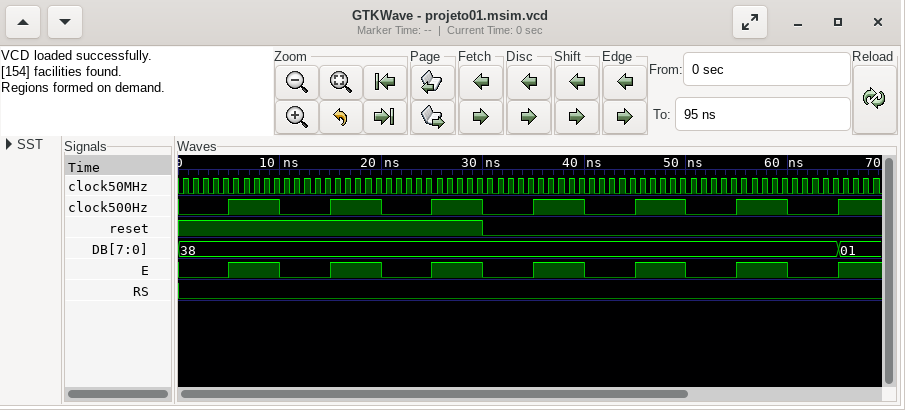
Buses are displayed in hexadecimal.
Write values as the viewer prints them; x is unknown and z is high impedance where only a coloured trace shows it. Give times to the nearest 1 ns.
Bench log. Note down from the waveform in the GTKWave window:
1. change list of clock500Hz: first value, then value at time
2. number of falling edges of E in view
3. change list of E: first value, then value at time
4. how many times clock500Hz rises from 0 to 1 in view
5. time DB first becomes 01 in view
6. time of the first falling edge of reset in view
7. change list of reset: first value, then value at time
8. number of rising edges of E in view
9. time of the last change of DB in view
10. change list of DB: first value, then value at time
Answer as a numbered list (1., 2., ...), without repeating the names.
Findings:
1. 0, 1 at 5 ns, 0 at 10 ns, 1 at 15 ns, 0 at 20 ns, 1 at 25 ns, 0 at 30 ns, 1 at 35 ns, 0 at 40 ns, 1 at 45 ns, 0 at 50 ns, 1 at 55 ns, 0 at 60 ns, 1 at 65 ns
2. 6
3. 0, 1 at 5 ns, 0 at 10 ns, 1 at 15 ns, 0 at 20 ns, 1 at 25 ns, 0 at 30 ns, 1 at 35 ns, 0 at 40 ns, 1 at 45 ns, 0 at 50 ns, 1 at 55 ns, 0 at 60 ns, 1 at 65 ns
4. 7
5. 65 ns
6. 30 ns
7. 1, 0 at 30 ns
8. 7
9. 65 ns
10. 38, 01 at 65 ns
